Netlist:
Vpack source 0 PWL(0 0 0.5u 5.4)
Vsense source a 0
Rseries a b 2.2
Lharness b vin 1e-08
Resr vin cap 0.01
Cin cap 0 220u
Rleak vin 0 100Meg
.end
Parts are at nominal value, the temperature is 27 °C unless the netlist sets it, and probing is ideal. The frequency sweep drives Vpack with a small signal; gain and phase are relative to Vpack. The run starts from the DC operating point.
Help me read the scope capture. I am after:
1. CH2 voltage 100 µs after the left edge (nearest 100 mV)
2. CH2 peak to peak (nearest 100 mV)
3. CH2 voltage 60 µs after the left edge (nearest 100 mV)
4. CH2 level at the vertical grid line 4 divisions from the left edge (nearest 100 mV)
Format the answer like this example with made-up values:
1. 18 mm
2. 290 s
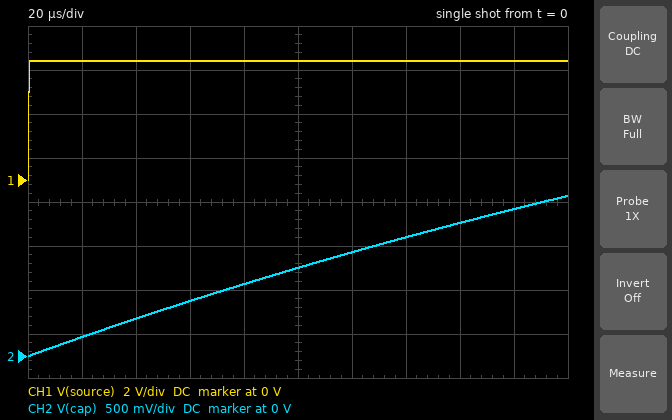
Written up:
1. 1.0 V
2. 1.8 V
3. 600 mV
4. 800 mV
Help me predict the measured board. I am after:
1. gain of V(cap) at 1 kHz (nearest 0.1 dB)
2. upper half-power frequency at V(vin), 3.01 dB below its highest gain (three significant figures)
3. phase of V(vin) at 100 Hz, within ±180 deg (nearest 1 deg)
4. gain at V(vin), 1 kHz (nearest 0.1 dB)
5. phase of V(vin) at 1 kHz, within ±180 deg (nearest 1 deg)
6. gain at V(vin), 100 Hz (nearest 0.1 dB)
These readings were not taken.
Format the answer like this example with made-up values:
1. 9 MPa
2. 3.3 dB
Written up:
1. -10.1 dB
2. 327 Hz
3. -17 deg
4. -10.1 dB
5. -71 deg
6. -0.4 dB
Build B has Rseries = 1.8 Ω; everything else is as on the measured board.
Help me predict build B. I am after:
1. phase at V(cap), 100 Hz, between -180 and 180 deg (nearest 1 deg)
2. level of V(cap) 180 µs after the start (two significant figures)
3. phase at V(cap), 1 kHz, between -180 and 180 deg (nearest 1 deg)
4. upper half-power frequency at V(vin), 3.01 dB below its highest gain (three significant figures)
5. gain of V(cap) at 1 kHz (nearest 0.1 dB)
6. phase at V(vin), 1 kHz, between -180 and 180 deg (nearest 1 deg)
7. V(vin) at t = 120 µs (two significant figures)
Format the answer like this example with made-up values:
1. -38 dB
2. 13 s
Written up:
1. -14 deg
2. 2.0 V
3. -68 deg
4. 400 Hz
5. -8.6 dB
6. -67 deg
7. 1.4 V
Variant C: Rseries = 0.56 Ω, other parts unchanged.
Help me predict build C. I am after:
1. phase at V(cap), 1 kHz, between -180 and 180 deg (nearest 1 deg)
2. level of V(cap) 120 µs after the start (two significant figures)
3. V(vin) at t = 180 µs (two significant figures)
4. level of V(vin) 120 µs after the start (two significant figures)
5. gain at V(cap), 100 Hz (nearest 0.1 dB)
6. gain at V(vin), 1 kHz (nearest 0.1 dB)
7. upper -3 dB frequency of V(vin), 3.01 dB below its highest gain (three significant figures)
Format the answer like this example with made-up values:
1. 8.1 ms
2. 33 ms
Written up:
1. -38 deg
2. 3.3 V
3. 4.1 V
4. 3.4 V
5. 0 dB
6. -2.1 dB
7. 1.27 kHz
